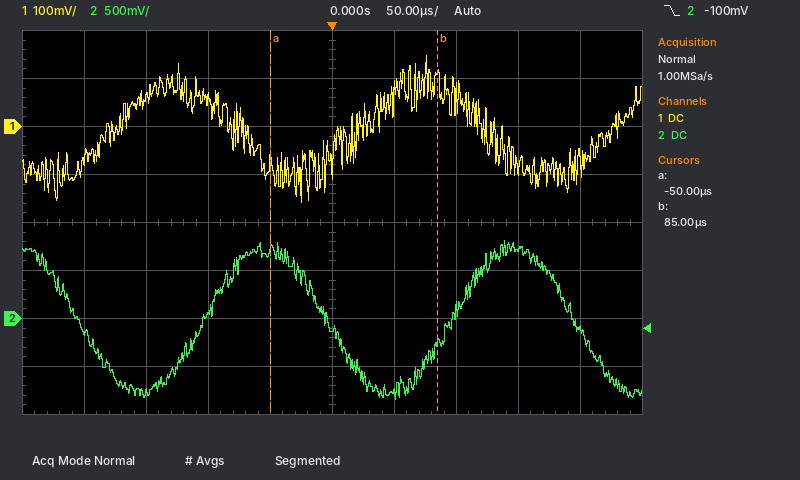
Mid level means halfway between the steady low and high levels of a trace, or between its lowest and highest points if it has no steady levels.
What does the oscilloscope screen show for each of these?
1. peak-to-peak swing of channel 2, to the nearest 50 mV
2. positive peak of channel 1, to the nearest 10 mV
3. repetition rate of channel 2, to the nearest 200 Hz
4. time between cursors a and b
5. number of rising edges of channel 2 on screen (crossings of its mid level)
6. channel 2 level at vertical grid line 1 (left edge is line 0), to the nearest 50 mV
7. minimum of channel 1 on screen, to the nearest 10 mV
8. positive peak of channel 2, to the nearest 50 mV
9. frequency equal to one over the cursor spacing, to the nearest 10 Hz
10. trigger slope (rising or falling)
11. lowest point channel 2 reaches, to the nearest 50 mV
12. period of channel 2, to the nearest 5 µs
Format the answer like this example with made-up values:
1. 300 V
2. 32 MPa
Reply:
1. 1.65 V
2. 150 mV
3. 5.0 kHz
4. 135 µs
5. 2
6. -150 mV
7. -160 mV
8. 800 mV
9. 7.41 kHz
10. falling
11. -850 mV
12. 200 µs
